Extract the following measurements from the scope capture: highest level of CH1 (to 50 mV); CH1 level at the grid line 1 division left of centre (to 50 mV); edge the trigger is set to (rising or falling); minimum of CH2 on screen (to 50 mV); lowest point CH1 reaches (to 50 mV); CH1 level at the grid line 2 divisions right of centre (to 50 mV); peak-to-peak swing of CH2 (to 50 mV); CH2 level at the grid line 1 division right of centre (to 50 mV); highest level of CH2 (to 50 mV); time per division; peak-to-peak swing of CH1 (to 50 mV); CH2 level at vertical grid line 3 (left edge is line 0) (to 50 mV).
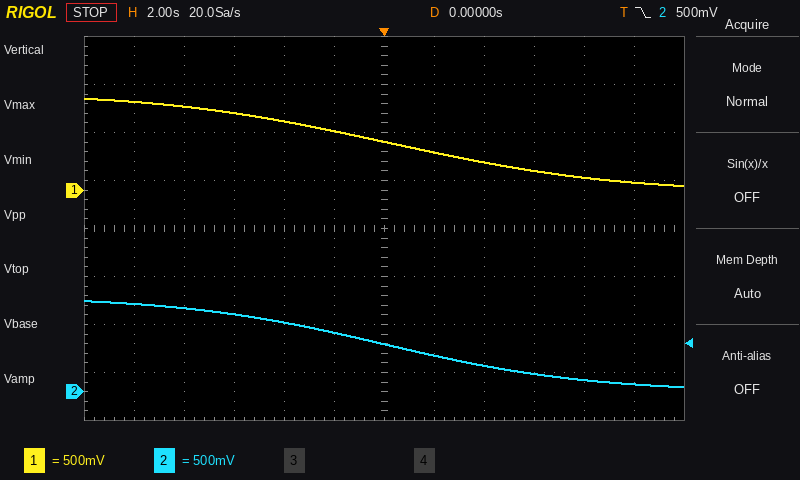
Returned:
950 mV
600 mV
falling
50 mV
50 mV
300 mV
900 mV
400 mV
950 mV
2 s
900 mV
800 mV
